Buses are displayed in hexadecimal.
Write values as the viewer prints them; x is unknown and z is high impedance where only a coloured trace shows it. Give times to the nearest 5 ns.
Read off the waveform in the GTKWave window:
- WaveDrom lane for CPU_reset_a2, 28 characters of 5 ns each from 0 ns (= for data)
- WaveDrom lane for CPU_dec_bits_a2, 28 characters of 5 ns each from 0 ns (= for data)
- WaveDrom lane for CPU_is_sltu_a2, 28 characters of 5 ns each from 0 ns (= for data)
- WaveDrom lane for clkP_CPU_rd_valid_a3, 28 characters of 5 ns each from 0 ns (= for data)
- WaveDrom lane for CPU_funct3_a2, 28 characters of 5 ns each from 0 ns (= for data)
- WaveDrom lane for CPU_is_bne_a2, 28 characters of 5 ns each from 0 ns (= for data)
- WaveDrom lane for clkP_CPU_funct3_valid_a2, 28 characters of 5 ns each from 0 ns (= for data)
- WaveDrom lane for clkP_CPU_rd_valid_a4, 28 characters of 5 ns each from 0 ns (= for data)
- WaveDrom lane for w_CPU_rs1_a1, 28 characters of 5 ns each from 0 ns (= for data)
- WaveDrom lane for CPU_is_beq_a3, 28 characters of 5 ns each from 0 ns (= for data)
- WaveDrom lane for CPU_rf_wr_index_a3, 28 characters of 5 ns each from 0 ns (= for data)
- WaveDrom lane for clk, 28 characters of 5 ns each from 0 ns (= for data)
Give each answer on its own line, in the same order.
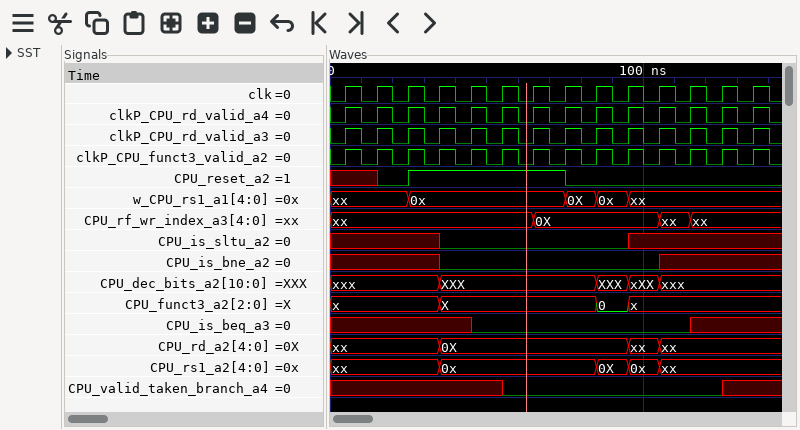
{name: 'CPU_reset_a2', wave: 'x..0.1.........0............'}
{name: 'CPU_dec_bits_a2', wave: 'x......=.........=.=.x......', data: 'XXX XXX xXX'}
{name: 'CPU_is_sltu_a2', wave: 'x......0...........x........'}
{name: 'clkP_CPU_rd_valid_a3', wave: '0101010101010101010101010101'}
{name: 'CPU_funct3_a2', wave: 'x......=.........=.x........', data: 'X 0'}
{name: 'CPU_is_bne_a2', wave: 'x......0.............x......'}
{name: 'clkP_CPU_funct3_valid_a2', wave: '0101010101010101010101010101'}
{name: 'clkP_CPU_rd_valid_a4', wave: '0101010101010101010101010101'}
{name: 'w_CPU_rs1_a1', wave: 'x....=.........=.=.x........', data: '0x 0X 0x'}
{name: 'CPU_is_beq_a3', wave: 'x........0.............x....'}
{name: 'CPU_rf_wr_index_a3', wave: 'x............=.......=.x....', data: '0X xx'}
{name: 'clk', wave: '0101010101010101010101010101'}
